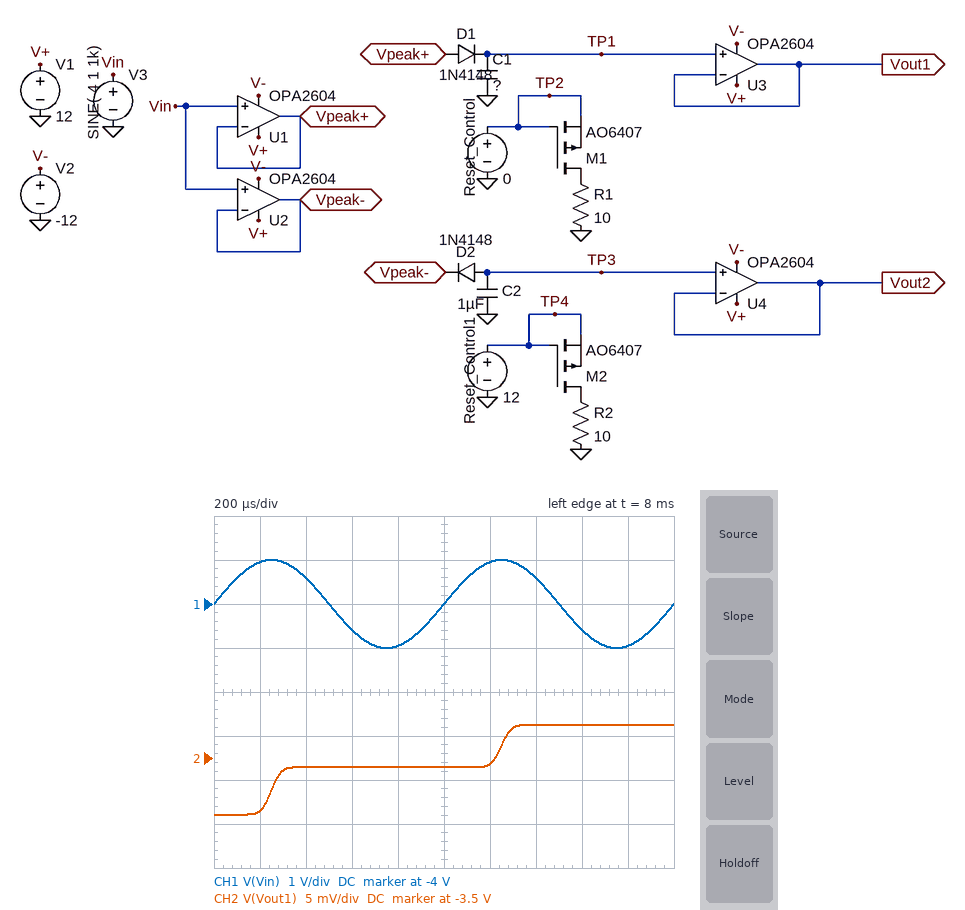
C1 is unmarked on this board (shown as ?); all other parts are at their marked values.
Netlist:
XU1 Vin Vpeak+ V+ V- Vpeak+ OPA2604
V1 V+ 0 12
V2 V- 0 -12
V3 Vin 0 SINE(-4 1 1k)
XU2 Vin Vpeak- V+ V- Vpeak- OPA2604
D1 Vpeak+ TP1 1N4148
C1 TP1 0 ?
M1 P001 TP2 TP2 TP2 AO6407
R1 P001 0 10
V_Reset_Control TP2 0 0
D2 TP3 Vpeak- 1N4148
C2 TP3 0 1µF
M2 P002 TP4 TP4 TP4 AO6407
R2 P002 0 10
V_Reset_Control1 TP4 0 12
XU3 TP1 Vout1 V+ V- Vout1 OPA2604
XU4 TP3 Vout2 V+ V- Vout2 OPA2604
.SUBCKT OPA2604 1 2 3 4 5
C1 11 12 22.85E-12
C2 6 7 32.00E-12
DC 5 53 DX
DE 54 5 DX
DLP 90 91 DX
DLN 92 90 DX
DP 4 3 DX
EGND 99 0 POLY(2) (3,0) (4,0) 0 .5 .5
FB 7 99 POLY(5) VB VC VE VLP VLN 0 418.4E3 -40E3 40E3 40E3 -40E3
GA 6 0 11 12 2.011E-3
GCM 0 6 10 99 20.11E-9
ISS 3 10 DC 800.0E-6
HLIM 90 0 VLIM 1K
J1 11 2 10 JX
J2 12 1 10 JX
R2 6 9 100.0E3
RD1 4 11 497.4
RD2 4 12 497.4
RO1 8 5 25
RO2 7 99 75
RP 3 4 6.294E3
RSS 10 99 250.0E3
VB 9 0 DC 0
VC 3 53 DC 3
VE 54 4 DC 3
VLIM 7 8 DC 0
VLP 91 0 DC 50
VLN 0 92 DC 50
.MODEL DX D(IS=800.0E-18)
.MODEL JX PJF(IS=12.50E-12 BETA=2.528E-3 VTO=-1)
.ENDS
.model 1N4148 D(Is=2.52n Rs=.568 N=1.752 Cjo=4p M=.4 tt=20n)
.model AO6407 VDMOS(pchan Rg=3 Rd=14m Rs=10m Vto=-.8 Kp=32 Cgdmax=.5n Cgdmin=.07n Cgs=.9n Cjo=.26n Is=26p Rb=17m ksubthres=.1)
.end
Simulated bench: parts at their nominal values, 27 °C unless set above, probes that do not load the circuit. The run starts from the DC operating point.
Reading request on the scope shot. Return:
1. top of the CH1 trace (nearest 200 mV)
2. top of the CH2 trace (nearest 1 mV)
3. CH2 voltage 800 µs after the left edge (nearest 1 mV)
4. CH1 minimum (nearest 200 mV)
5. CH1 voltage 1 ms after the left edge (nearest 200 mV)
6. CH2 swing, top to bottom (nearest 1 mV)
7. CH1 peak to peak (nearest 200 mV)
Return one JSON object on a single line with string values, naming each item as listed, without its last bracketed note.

{"top of the CH1 trace": "-3.0 V", "top of the CH2 trace": "-3.496 V", "CH2 voltage 800 µs after the left edge": "-3.501 V", "CH1 minimum": "-5.0 V", "CH1 voltage 1 ms after the left edge": "-4.0 V", "CH2 swing, top to bottom": "10 mV", "CH1 peak to peak": "2.0 V"}
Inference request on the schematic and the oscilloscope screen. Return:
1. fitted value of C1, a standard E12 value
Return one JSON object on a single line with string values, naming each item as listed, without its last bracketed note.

{"fitted value of C1, a standard E12 value": "2.7 µF"}
